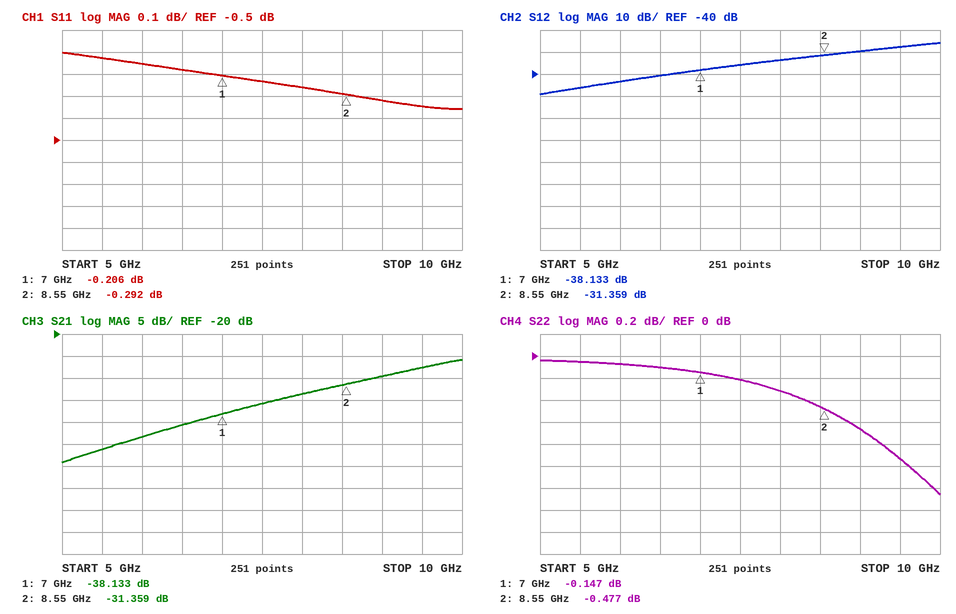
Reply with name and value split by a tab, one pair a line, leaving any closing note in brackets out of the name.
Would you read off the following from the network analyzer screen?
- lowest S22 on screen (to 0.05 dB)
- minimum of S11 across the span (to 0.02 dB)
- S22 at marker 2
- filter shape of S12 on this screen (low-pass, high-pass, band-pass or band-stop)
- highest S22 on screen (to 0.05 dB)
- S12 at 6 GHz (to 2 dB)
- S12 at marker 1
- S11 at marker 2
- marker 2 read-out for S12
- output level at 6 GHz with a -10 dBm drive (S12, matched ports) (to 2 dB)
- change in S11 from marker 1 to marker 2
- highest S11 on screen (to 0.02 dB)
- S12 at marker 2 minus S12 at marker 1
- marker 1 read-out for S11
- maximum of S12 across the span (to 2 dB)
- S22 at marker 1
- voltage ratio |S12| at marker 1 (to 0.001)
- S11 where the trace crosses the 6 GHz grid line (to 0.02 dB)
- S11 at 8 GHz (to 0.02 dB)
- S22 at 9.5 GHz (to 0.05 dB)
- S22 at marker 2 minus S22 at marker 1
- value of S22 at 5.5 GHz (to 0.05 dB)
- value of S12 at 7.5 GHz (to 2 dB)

lowest S22 on screen	-1.25 dB
minimum of S11 across the span	-0.36 dB
S22 at marker 2	-0.477 dB
filter shape of S12 on this screen	high-pass
highest S22 on screen	-0.05 dB
S12 at 6 GHz	-44 dB
S12 at marker 1	-38.133 dB
S11 at marker 2	-0.292 dB
marker 2 read-out for S12	-31.359 dB
output level at 6 GHz with a -10 dBm drive (S12, matched ports)	-54 dBm
change in S11 from marker 1 to marker 2	-0.086 dB
highest S11 on screen	-0.10 dB
S12 at marker 2 minus S12 at marker 1	6.774 dB
marker 1 read-out for S11	-0.206 dB
maximum of S12 across the span	-26 dB
S22 at marker 1	-0.147 dB
voltage ratio |S12| at marker 1	0.012
S11 where the trace crosses the 6 GHz grid line	-0.16 dB
S11 at 8 GHz	-0.26 dB
S22 at 9.5 GHz	-0.95 dB
S22 at marker 2 minus S22 at marker 1	-0.330 dB
value of S22 at 5.5 GHz	-0.05 dB
value of S12 at 7.5 GHz	-36 dB
